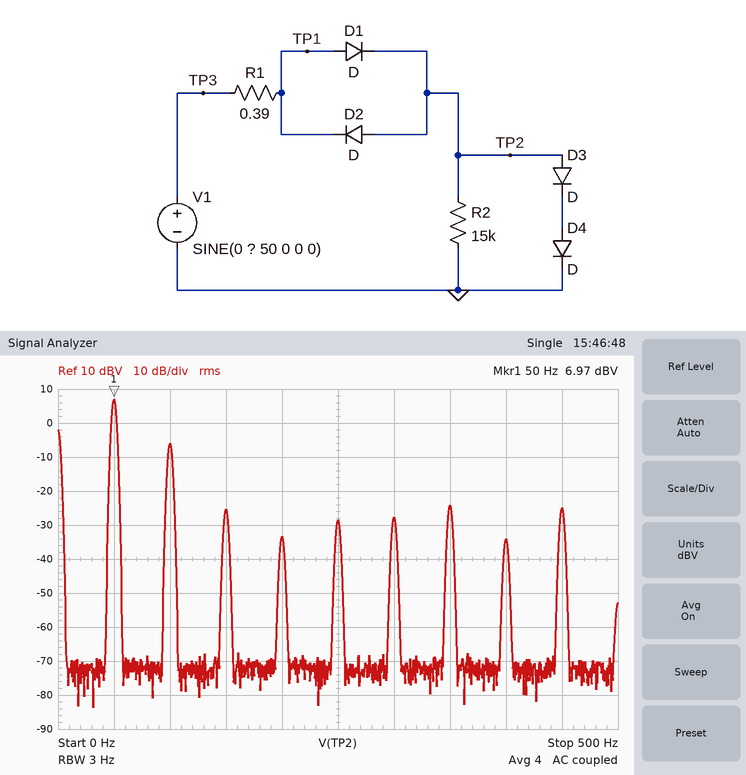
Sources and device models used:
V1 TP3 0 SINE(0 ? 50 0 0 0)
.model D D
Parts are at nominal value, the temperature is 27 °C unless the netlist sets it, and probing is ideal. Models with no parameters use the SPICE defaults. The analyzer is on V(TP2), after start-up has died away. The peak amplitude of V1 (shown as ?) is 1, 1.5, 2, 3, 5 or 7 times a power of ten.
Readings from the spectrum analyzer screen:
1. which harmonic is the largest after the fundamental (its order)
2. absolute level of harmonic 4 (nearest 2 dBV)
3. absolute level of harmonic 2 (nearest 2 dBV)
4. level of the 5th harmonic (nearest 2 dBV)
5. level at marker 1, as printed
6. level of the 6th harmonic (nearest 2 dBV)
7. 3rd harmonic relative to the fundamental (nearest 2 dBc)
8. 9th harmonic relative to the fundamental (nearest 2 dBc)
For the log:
2
-34 dBV
-6 dBV
-28 dBV
6.97 dBV
-28 dBV
-32 dBc
-32 dBc
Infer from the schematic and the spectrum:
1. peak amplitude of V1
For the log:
5 V
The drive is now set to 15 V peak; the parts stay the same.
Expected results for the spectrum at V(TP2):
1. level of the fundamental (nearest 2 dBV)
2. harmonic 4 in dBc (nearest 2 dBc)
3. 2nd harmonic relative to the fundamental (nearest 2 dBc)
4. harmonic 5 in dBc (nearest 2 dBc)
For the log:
16 dBV
-24 dBc
-8 dBc
-38 dBc
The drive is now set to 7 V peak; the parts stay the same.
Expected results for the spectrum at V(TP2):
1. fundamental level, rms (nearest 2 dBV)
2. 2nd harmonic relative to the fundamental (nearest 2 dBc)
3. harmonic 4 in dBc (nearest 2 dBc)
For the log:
10 dBV
-10 dBc
-34 dBc
